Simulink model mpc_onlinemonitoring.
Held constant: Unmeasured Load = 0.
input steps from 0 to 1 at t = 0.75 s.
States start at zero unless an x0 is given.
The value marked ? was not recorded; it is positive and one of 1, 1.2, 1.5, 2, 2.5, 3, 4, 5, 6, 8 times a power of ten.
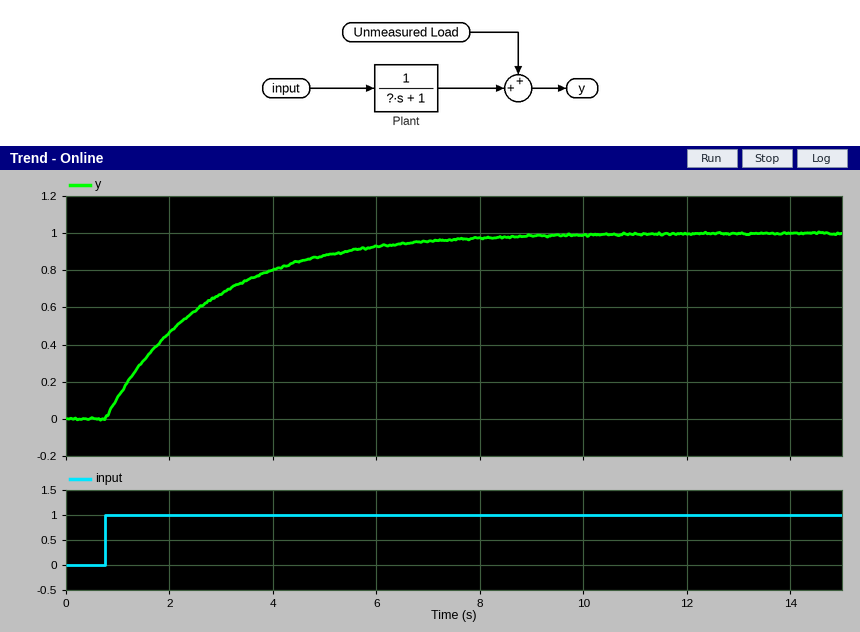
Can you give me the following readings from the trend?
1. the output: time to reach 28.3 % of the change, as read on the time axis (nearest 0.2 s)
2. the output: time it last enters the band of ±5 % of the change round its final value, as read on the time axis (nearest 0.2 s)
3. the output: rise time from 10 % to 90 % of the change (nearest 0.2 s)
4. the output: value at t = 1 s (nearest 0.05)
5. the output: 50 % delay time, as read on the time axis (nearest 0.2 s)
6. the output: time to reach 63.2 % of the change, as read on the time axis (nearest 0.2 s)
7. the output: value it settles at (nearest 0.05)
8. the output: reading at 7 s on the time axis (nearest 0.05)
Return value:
1.4 s
6.8 s
4.4 s
0.10
2.2 s
2.8 s
1.00
0.95
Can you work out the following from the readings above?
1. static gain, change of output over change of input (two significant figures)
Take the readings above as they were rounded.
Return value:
1.0
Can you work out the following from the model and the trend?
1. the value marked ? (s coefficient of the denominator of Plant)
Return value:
2
